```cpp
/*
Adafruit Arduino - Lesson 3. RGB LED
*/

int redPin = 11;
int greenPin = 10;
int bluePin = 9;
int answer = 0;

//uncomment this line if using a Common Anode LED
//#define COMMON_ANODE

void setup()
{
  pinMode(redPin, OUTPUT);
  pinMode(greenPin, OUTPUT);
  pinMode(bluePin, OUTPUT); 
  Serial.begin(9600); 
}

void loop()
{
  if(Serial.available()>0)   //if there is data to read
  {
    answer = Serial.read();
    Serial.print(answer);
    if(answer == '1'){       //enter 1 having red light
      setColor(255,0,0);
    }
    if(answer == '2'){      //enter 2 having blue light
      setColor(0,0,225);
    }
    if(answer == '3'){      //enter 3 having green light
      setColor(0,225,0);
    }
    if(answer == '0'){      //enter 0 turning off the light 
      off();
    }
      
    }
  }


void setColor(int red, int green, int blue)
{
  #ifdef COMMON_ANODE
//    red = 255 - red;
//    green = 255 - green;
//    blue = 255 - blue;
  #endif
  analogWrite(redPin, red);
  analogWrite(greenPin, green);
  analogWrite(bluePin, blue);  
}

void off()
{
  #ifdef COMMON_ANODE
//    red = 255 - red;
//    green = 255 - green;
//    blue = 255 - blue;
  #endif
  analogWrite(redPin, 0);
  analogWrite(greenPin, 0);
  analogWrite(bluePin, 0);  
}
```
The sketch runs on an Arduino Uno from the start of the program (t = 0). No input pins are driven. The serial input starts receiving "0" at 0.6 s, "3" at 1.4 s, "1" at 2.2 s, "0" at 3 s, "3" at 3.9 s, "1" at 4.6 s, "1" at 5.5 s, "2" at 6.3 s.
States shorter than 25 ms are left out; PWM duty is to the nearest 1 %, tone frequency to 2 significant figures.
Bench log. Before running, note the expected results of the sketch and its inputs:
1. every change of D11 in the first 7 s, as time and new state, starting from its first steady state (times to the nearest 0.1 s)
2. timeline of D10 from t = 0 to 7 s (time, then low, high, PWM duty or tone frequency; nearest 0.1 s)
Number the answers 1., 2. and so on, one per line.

1. 0 s low; 2.2 s high; 3 s low; 4.6 s high; 6.3 s low
2. 0 s low; 1.4 s PWM 88 %; 2.2 s low; 3.9 s PWM 88 %; 4.6 s low
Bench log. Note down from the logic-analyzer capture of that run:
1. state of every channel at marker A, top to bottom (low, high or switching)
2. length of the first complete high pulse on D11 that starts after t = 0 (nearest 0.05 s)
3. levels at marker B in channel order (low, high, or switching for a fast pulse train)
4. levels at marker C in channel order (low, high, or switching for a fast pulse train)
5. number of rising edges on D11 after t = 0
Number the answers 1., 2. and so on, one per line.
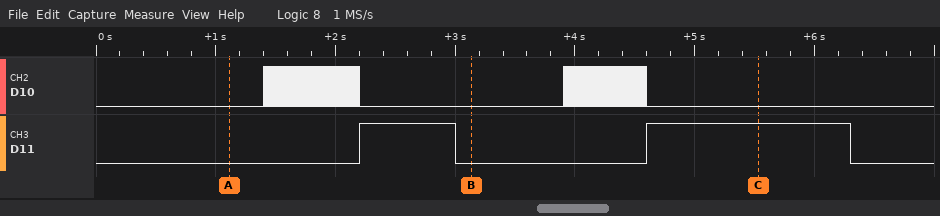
1. D10 low, D11 low
2. 0.80 s
3. D10 low, D11 low
4. D10 low, D11 high
5. 2
